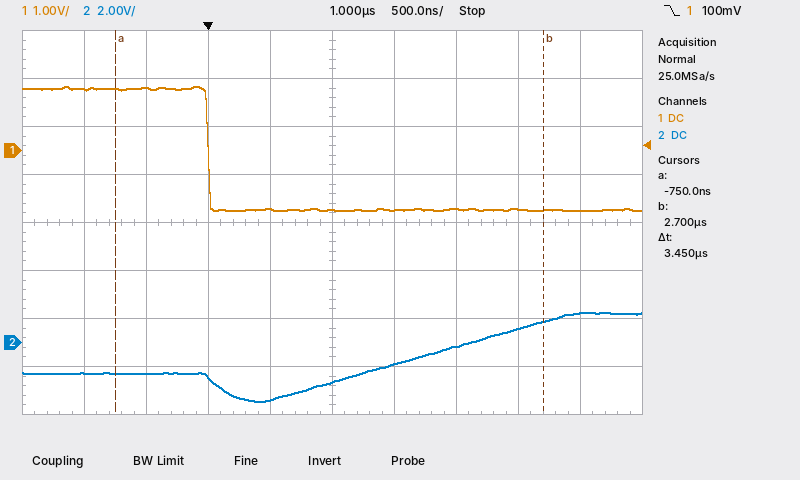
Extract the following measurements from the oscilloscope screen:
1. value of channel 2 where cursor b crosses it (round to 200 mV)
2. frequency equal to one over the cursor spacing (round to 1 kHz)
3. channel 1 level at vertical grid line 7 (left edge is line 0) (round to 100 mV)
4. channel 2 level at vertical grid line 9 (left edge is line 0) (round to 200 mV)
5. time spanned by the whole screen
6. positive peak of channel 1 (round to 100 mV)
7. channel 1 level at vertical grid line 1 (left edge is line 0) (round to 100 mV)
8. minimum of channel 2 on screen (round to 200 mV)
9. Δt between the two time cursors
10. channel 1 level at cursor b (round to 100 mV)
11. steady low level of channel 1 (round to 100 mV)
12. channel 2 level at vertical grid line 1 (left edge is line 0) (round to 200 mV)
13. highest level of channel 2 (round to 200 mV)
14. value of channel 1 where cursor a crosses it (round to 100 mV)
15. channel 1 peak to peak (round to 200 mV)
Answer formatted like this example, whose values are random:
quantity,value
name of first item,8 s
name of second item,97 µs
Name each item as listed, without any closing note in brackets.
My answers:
quantity,value
value of channel 2 where cursor b crosses it,800 mV
frequency equal to one over the cursor spacing,290 kHz
channel 1 level at vertical grid line 7 (left edge is line 0),-1.2 V
channel 2 level at vertical grid line 9 (left edge is line 0),1.2 V
time spanned by the whole screen,5 µs
positive peak of channel 1,1.3 V
channel 1 level at vertical grid line 1 (left edge is line 0),1.3 V
minimum of channel 2 on screen,-2.4 V
Δt between the two time cursors,3.45 µs
channel 1 level at cursor b,-1.2 V
steady low level of channel 1,-1.2 V
channel 2 level at vertical grid line 1 (left edge is line 0),-1.2 V
highest level of channel 2,1.2 V
value of channel 1 where cursor a crosses it,1.3 V
channel 1 peak to peak,2.6 V
